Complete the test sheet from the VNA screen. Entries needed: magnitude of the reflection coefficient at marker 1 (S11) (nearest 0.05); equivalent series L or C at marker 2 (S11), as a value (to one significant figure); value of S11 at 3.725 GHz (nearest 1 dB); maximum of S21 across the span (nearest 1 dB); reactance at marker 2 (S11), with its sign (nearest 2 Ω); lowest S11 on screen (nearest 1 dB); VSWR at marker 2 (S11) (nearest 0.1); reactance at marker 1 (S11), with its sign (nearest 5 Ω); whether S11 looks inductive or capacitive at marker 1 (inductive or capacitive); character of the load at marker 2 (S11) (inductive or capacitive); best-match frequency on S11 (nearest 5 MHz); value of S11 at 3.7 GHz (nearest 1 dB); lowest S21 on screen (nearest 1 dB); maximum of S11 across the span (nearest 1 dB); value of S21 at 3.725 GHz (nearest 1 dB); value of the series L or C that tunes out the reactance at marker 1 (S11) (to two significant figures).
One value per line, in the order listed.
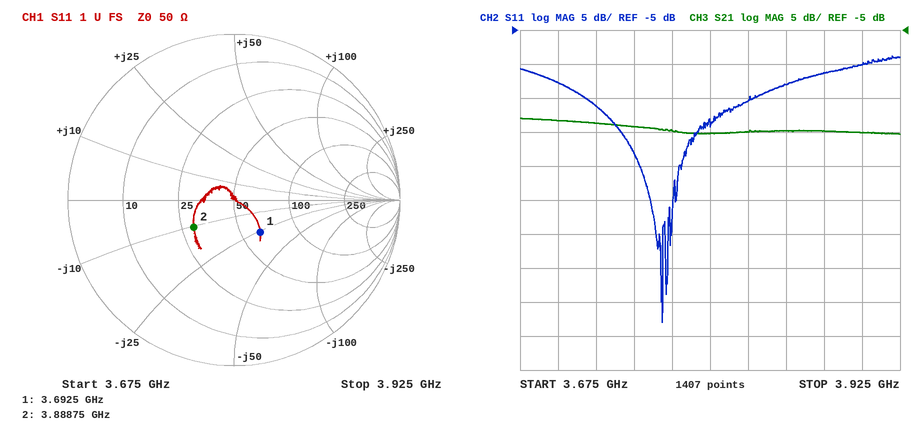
0.25
4 pF
-16 dB
-18 dB
-10 Ω
-48 dB
1.8
-25 Ω
capacitive
capacitive
3.770 GHz
-13 dB
-20 dB
-9 dB
-19 dB
1.1 nH
